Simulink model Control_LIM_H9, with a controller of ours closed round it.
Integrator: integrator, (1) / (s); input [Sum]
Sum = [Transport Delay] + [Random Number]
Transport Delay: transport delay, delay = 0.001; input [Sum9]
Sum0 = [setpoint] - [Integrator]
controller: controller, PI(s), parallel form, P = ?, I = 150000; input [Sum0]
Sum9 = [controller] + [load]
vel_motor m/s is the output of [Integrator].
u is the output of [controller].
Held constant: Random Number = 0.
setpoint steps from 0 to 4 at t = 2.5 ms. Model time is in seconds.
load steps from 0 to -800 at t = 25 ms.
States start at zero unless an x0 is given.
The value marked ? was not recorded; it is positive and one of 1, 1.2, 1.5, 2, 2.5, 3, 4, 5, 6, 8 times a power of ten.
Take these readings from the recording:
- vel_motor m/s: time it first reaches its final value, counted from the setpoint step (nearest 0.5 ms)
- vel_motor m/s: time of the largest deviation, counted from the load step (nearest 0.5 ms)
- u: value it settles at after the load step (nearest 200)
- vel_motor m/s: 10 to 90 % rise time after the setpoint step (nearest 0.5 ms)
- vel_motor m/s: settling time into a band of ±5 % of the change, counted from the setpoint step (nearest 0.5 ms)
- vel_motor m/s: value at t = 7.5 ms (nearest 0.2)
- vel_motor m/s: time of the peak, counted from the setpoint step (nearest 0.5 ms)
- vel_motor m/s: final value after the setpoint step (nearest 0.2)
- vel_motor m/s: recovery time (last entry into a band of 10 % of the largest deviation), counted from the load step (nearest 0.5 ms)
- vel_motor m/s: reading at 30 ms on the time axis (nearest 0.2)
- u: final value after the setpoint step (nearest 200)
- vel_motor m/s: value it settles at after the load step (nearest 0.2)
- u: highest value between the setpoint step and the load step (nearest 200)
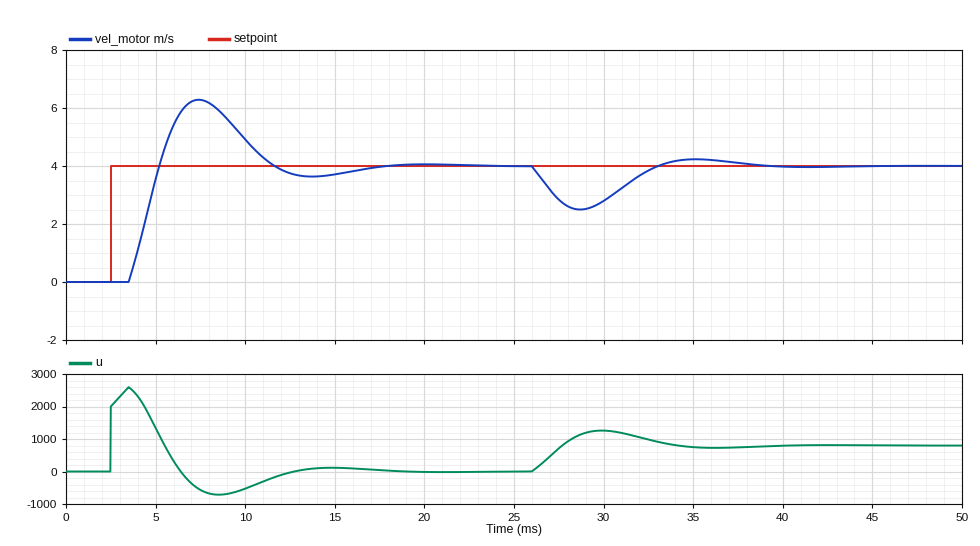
2.5 ms
3.5 ms
800
1.5 ms
13.5 ms
6.2
5.0 ms
4.0
12.0 ms
2.8
0
4.0
2600
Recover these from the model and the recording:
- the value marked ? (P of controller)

500
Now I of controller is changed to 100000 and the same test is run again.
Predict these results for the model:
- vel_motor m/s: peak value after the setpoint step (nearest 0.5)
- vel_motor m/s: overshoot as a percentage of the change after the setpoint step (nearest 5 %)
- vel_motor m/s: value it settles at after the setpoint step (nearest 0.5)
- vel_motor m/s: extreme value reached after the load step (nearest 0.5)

5.5
40 %
4.0
2.5
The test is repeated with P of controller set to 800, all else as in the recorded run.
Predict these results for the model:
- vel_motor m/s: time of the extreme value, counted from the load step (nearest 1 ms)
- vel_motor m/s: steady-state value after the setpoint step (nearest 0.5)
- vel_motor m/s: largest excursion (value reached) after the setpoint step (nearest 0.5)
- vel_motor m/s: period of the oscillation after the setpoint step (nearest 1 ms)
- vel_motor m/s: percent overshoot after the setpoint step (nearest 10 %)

3 ms
4.0
6.5
6 ms
60 %
